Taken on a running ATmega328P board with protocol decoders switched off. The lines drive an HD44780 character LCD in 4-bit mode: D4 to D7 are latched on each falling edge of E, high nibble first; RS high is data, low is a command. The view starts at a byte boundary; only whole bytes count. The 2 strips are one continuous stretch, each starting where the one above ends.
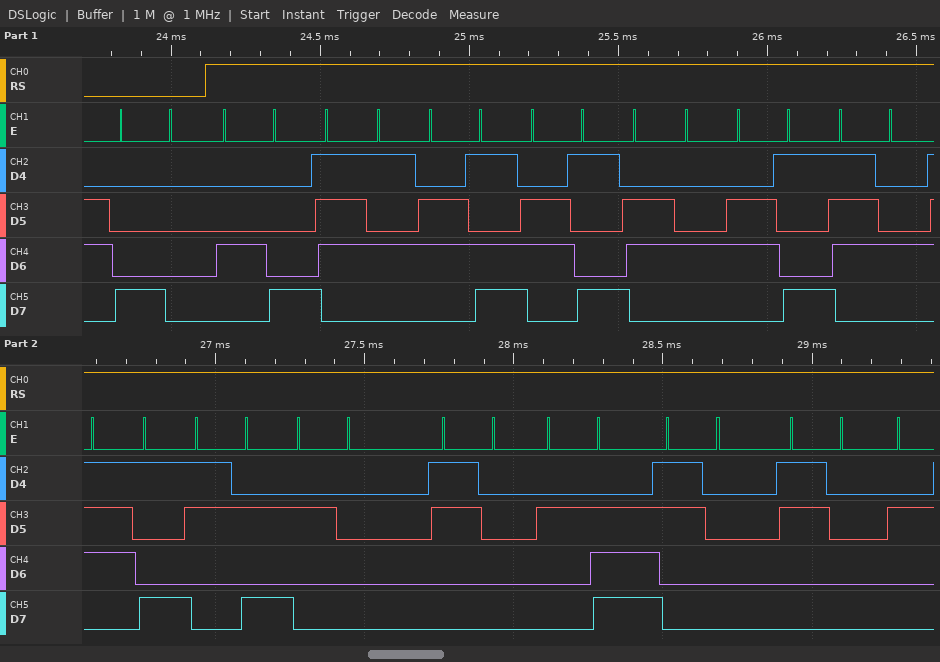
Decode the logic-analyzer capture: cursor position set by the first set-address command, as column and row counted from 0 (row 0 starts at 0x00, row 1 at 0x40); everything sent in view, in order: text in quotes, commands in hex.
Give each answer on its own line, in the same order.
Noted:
column 0, row 0
0x80 "Humidity: 0.00"
